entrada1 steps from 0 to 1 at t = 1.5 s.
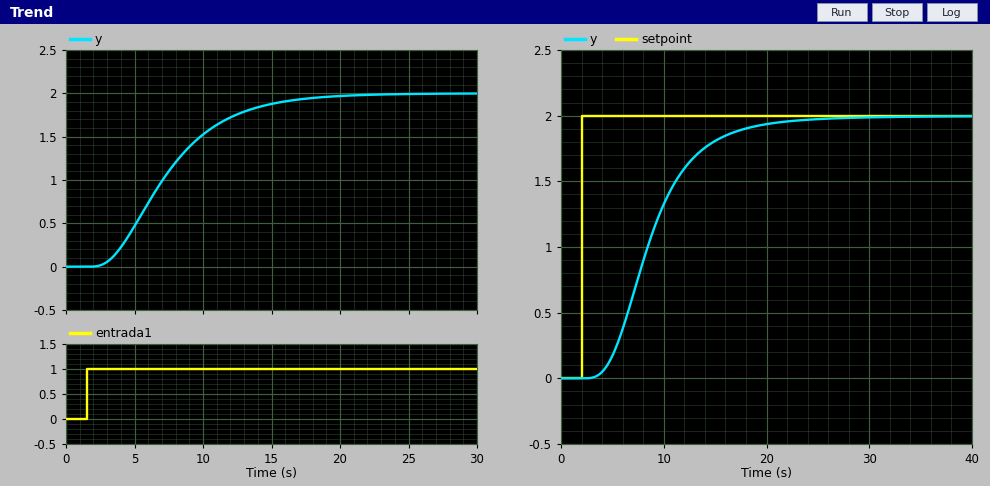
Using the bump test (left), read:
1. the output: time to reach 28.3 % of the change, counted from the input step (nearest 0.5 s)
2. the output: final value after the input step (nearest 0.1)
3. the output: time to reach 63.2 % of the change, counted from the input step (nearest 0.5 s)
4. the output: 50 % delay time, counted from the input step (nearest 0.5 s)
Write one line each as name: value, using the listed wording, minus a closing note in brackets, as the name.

the output: time to reach 28.3 % of the change, counted from the input step: 4.0 s
the output: final value after the input step: 2.0
the output: time to reach 63.2 % of the change, counted from the input step: 7.0 s
the output: 50 % delay time, counted from the input step: 5.5 s
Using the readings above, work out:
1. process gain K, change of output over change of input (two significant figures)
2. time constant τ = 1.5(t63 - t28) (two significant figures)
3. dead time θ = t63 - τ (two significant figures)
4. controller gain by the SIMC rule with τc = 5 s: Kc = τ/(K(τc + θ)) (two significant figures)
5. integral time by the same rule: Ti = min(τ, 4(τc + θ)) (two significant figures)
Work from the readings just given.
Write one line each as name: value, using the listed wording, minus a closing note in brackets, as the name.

process gain K, change of output over change of input: 2.0
time constant τ = 1.5(t63 - t28): 4.5 s
dead time θ = t63 - τ: 2.5 s
controller gain by the SIMC rule with τc = 5 s: Kc = τ/(K(τc + θ)): 0.30
integral time by the same rule: Ti = min(τ, 4(τc + θ)): 4.5 s
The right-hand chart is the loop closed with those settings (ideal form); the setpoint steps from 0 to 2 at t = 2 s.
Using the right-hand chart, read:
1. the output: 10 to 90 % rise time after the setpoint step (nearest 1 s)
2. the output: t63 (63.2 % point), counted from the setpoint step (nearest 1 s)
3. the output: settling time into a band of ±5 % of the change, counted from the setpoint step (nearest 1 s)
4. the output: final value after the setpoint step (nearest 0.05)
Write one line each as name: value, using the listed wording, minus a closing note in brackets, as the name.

the output: 10 to 90 % rise time after the setpoint step: 10 s
the output: t63 (63.2 % point), counted from the setpoint step: 8 s
the output: settling time into a band of ±5 % of the change, counted from the setpoint step: 16 s
the output: final value after the setpoint step: 2.00
